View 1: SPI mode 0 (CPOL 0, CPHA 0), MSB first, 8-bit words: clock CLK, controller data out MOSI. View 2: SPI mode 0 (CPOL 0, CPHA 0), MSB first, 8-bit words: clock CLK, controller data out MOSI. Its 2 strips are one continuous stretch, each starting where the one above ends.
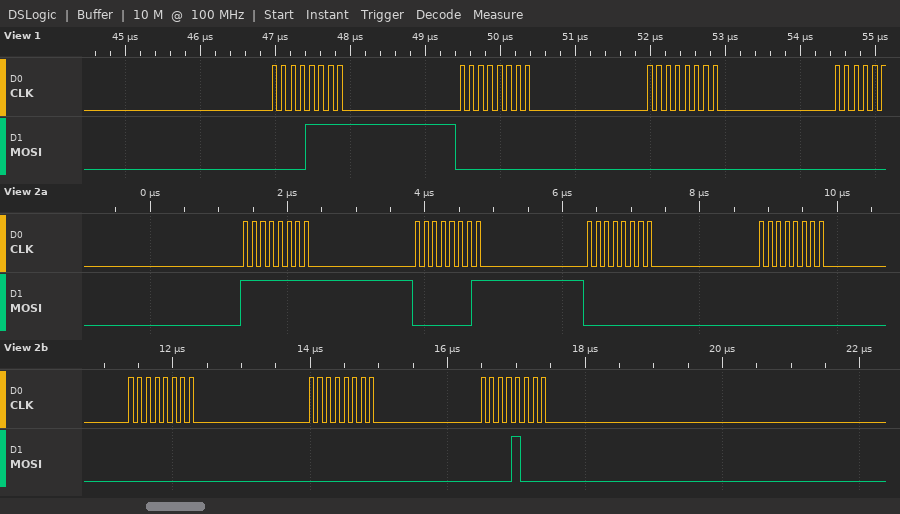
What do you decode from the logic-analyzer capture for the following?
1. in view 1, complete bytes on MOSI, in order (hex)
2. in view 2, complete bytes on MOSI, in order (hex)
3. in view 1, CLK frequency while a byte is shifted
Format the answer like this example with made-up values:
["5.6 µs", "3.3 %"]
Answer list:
["0F 00 00", "FF 01 00 00 00 00 08", "8 MHz"]
